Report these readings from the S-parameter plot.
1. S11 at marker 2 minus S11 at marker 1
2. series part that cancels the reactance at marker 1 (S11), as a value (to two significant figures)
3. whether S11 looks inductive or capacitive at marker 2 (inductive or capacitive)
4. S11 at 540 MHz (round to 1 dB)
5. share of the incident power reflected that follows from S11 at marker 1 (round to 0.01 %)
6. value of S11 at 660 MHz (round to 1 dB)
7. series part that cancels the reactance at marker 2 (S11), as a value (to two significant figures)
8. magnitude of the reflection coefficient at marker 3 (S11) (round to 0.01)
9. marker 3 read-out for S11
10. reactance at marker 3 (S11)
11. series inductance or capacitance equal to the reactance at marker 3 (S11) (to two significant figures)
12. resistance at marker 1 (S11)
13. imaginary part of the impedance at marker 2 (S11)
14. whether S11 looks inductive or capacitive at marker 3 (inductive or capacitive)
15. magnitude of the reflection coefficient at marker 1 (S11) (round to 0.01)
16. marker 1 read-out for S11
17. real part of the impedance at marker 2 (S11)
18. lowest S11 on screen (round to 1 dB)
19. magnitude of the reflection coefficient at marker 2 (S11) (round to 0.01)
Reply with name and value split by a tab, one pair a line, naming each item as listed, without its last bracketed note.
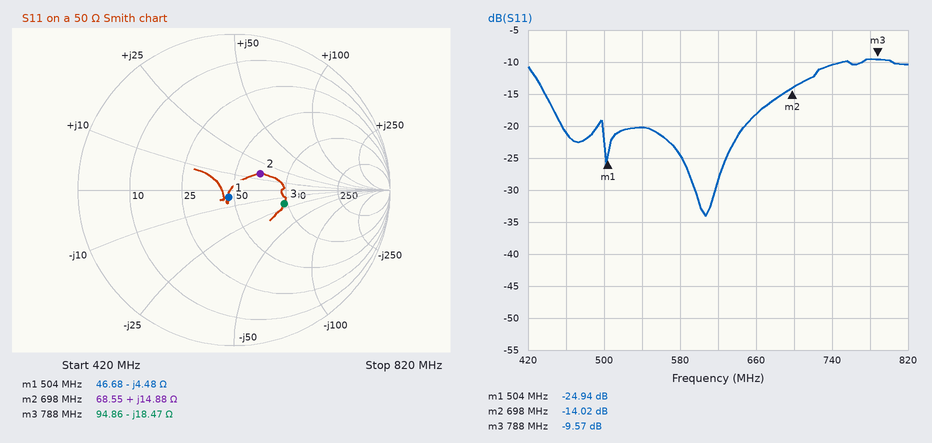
S11 at marker 2 minus S11 at marker 1	10.92 dB
series part that cancels the reactance at marker 1 (S11), as a value	1.4 nH
whether S11 looks inductive or capacitive at marker 2	inductive
S11 at 540 MHz	-20 dB
share of the incident power reflected that follows from S11 at marker 1	0.32 %
value of S11 at 660 MHz	-18 dB
series part that cancels the reactance at marker 2 (S11), as a value	15 pF
magnitude of the reflection coefficient at marker 3 (S11)	0.33
marker 3 read-out for S11	-9.57 dB
reactance at marker 3	-18.47 Ω
series inductance or capacitance equal to the reactance at marker 3 (S11)	11 pF
resistance at marker 1	46.68 Ω
imaginary part of the impedance at marker 2	+14.88 Ω
whether S11 looks inductive or capacitive at marker 3	capacitive
magnitude of the reflection coefficient at marker 1 (S11)	0.06
marker 1 read-out for S11	-24.94 dB
real part of the impedance at marker 2	68.55 Ω
lowest S11 on screen	-34 dB
magnitude of the reflection coefficient at marker 2 (S11)	0.20
